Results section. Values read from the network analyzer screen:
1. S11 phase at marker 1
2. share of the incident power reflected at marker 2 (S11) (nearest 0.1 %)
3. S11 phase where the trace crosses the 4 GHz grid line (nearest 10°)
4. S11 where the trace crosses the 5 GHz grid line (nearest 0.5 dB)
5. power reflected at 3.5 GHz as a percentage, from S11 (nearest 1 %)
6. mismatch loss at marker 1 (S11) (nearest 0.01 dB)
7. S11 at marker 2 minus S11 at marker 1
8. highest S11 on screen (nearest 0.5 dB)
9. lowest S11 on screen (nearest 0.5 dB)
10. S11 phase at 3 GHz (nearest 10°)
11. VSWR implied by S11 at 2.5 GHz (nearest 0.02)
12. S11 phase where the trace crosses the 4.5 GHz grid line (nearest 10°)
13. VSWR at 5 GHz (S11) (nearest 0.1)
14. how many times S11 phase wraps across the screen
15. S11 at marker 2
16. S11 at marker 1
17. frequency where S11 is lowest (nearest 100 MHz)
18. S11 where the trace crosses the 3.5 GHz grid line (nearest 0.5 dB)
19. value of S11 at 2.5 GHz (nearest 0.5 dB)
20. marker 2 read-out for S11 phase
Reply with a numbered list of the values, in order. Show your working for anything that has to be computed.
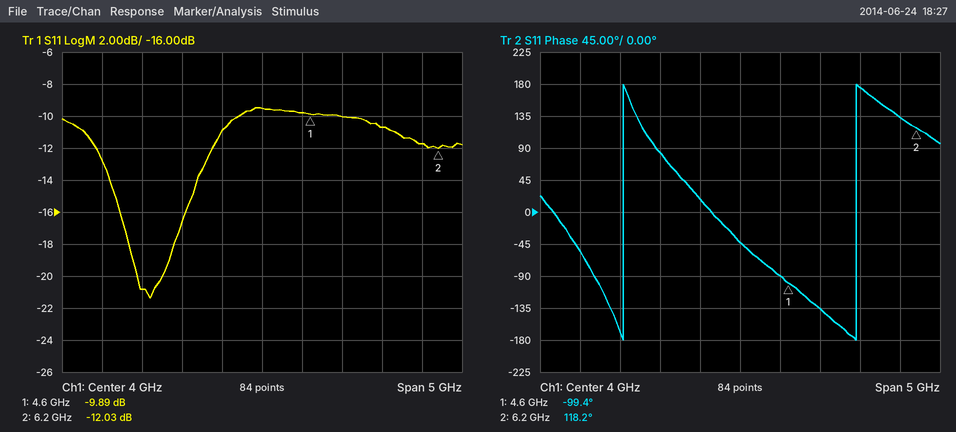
1. -99.4°
2. 10^(-12.03/10) ≈ 6.3 %
3. -40°
4. -10.0 dB
5. 10^(-11/10) ≈ 8 %
6. −10 log10(1 − 10^(-9.89/10)) ≈ 0.47 dB
7. -12.03 − (-9.89) = -2.14 dB
8. -9.5 dB
9. -21.5 dB
10. 80°
11. |Γ| = 10^(-21/20) = 0.0891; VSWR = (1 + 0.0891)/(1 − 0.0891) ≈ 1.20
12. -90°
13. |Γ| = 10^(-10/20) = 0.3162; VSWR = (1 + 0.3162)/(1 − 0.3162) ≈ 1.9
14. 2
15. -12.03 dB
16. -9.89 dB
17. 2.6 GHz
18. -11.0 dB
19. -21.0 dB
20. 118.2°
